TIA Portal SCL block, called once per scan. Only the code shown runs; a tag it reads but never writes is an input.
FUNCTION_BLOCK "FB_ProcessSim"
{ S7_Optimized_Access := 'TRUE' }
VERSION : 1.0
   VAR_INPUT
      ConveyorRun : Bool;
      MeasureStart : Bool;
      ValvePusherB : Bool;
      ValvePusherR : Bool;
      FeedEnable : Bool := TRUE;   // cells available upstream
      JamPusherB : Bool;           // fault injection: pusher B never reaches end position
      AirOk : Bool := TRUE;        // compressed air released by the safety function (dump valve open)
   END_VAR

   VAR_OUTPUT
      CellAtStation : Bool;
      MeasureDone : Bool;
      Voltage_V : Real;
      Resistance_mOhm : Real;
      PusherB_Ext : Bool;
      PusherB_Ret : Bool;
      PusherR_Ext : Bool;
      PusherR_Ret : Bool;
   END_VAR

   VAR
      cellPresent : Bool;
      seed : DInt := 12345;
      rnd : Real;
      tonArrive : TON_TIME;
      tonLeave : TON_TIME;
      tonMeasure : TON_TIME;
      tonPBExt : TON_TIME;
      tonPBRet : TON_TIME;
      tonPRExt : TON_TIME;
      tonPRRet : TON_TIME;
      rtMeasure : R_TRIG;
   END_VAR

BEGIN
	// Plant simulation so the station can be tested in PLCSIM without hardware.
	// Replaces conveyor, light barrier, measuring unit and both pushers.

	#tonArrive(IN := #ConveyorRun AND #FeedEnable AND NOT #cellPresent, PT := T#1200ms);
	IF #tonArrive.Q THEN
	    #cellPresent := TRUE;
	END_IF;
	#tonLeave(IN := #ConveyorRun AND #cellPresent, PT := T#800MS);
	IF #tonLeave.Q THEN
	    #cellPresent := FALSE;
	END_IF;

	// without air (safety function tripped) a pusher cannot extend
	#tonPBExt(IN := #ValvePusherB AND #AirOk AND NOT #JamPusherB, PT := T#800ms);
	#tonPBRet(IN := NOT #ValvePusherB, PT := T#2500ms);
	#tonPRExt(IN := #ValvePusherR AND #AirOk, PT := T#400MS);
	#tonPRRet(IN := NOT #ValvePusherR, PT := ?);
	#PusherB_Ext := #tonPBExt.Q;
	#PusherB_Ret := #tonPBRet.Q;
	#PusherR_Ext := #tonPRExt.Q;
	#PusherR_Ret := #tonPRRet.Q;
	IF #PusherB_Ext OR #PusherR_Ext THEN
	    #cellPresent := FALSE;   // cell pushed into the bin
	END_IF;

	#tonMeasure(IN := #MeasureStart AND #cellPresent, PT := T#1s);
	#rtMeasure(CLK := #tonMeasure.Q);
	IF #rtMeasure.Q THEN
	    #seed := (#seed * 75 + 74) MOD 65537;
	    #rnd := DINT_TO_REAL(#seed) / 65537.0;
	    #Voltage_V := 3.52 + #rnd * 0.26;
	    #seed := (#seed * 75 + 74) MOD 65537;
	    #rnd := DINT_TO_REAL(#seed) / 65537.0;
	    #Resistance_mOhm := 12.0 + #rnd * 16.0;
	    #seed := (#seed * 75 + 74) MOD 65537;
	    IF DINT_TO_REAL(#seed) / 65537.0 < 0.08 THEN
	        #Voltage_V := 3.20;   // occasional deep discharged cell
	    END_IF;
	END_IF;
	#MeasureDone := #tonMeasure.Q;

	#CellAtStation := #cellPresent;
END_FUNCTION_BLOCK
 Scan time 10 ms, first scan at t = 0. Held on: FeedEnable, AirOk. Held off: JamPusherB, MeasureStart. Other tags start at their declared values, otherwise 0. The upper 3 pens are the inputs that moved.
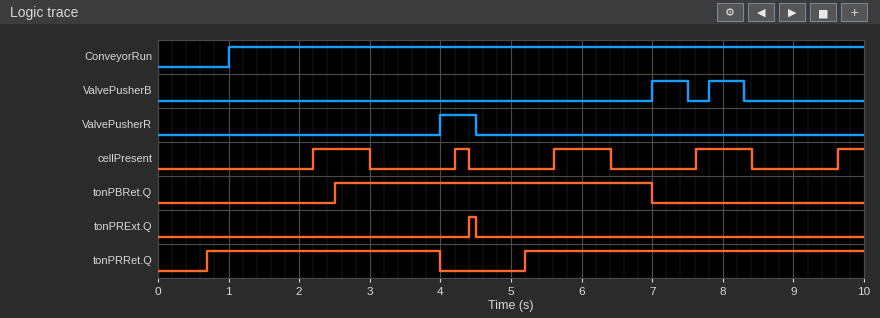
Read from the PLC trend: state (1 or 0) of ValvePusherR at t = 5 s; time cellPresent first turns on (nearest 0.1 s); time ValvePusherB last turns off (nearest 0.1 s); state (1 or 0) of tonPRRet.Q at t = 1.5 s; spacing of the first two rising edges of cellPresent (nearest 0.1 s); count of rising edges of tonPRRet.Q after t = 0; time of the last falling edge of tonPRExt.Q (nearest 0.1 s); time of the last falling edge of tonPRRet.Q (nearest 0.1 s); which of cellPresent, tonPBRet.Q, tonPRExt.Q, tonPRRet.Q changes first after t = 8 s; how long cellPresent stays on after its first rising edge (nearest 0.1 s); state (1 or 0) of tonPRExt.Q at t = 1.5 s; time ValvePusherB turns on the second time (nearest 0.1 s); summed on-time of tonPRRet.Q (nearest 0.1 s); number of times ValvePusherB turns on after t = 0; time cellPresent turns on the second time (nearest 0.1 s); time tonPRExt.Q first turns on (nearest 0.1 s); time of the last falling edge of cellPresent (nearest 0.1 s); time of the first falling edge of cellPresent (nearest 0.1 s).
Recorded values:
0
2.2 s
8.3 s
1
2.0 s
2
4.5 s
4.0 s
cellPresent
0.8 s
0
7.8 s
8.1 s
2
4.2 s
4.4 s
8.4 s
3.0 s
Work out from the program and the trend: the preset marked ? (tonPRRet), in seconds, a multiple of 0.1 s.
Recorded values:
0.7 s
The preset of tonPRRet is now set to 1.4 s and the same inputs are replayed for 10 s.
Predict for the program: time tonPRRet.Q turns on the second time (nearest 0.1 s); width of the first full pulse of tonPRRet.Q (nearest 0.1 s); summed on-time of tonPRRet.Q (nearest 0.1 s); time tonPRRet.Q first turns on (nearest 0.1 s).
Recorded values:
5.9 s
2.6 s
6.7 s
1.4 s
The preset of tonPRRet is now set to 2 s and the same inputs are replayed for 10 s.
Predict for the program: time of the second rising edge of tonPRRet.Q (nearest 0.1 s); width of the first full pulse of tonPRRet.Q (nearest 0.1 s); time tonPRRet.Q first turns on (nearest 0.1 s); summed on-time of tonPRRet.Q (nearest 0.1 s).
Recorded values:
6.5 s
2.0 s
2.0 s
5.5 s
